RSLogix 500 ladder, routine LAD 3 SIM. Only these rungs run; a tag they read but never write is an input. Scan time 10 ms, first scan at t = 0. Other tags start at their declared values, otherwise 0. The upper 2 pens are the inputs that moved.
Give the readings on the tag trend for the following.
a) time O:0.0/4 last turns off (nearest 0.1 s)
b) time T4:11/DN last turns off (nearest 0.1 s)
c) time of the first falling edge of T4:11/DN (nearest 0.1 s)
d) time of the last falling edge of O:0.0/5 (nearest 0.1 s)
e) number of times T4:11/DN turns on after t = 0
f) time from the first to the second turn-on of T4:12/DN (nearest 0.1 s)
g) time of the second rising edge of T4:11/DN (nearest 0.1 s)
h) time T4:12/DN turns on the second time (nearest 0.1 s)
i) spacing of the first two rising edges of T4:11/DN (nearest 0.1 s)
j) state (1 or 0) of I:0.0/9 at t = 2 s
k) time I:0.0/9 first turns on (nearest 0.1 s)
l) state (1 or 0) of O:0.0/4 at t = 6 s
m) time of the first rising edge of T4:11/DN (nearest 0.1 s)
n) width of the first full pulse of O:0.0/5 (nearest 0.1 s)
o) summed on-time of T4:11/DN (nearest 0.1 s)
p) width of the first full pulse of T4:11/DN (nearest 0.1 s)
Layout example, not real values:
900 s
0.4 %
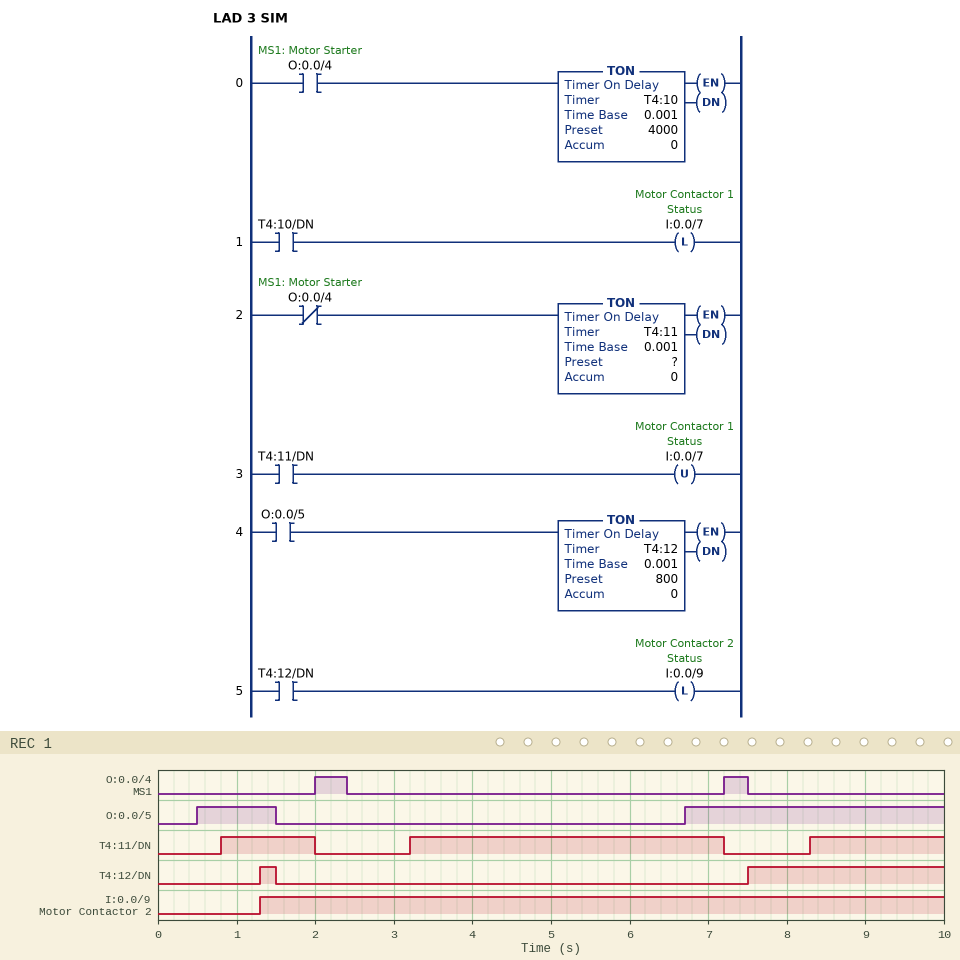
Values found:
7.5 s
7.2 s
2.0 s
1.5 s
3
6.2 s
3.2 s
7.5 s
2.4 s
1
1.3 s
0
0.8 s
1.0 s
6.9 s
1.2 s
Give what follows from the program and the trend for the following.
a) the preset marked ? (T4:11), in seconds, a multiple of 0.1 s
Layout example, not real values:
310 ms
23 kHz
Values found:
0.8 s
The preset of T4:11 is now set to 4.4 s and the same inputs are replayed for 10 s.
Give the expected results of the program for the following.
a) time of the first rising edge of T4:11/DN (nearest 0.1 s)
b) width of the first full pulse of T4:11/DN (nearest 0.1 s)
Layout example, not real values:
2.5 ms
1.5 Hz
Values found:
6.8 s
0.4 s
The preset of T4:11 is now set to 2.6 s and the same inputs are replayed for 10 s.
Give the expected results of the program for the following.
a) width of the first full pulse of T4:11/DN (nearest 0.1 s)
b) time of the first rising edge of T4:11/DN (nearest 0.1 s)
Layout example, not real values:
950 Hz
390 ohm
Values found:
2.2 s
5.0 s
